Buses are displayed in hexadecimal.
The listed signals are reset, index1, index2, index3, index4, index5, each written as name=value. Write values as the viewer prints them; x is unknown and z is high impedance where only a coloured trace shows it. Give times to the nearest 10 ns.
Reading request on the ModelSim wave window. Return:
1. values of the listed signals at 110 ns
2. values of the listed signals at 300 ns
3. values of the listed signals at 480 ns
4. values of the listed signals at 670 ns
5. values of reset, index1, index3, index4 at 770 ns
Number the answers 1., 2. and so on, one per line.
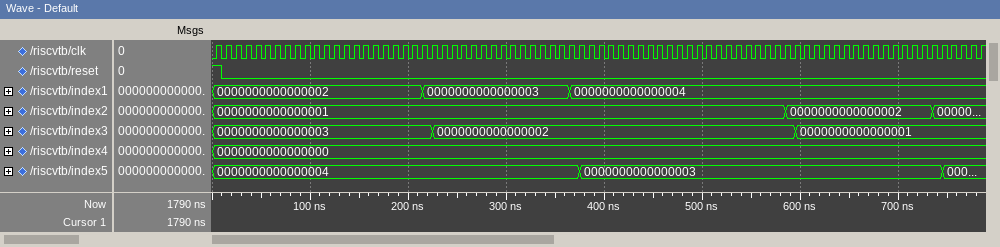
1. reset=0, index1=0000000000000002, index2=0000000000000001, index3=0000000000000003, index4=0000000000000000, index5=0000000000000004
2. reset=0, index1=0000000000000003, index2=0000000000000001, index3=0000000000000002, index4=0000000000000000, index5=0000000000000004
3. reset=0, index1=0000000000000004, index2=0000000000000001, index3=0000000000000002, index4=0000000000000000, index5=0000000000000003
4. reset=0, index1=0000000000000004, index2=0000000000000002, index3=0000000000000001, index4=0000000000000000, index5=0000000000000003
5. reset=0, index1=0000000000000004, index3=0000000000000001, index4=0000000000000000
